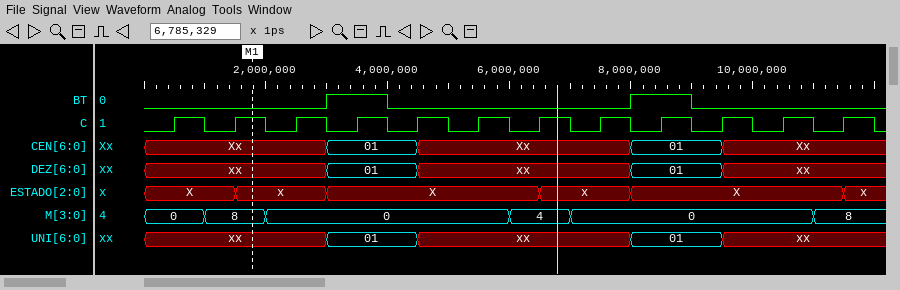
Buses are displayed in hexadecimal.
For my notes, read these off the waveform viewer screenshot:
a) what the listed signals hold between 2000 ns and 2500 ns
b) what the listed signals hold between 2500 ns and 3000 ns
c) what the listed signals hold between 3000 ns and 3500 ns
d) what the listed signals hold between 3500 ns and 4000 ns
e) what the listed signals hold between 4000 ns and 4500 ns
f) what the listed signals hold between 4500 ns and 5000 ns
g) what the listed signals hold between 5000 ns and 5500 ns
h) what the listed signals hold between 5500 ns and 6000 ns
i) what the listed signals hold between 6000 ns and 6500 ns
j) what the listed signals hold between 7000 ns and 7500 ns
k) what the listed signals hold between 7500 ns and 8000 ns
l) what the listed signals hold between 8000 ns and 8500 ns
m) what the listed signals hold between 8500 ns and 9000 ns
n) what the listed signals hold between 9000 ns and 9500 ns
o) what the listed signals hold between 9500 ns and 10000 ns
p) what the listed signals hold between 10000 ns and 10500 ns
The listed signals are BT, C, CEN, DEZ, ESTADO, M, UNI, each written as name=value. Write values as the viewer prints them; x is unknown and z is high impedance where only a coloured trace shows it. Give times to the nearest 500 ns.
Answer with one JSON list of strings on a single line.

["BT=0, C=0, CEN=Xx, DEZ=xx, ESTADO=x, M=0, UNI=xx", "BT=0, C=1, CEN=Xx, DEZ=xx, ESTADO=x, M=0, UNI=xx", "BT=1, C=0, CEN=01, DEZ=01, ESTADO=X, M=0, UNI=01", "BT=1, C=1, CEN=01, DEZ=01, ESTADO=X, M=0, UNI=01", "BT=0, C=0, CEN=01, DEZ=01, ESTADO=X, M=0, UNI=01", "BT=0, C=1, CEN=Xx, DEZ=xx, ESTADO=X, M=0, UNI=xx", "BT=0, C=0, CEN=Xx, DEZ=xx, ESTADO=X, M=0, UNI=xx", "BT=0, C=1, CEN=Xx, DEZ=xx, ESTADO=X, M=0, UNI=xx", "BT=0, C=0, CEN=Xx, DEZ=xx, ESTADO=X, M=4, UNI=xx", "BT=0, C=0, CEN=Xx, DEZ=xx, ESTADO=x, M=0, UNI=xx", "BT=0, C=1, CEN=Xx, DEZ=xx, ESTADO=x, M=0, UNI=xx", "BT=1, C=0, CEN=01, DEZ=01, ESTADO=X, M=0, UNI=01", "BT=1, C=1, CEN=01, DEZ=01, ESTADO=X, M=0, UNI=01", "BT=0, C=0, CEN=01, DEZ=01, ESTADO=X, M=0, UNI=01", "BT=0, C=1, CEN=Xx, DEZ=xx, ESTADO=X, M=0, UNI=xx", "BT=0, C=0, CEN=Xx, DEZ=xx, ESTADO=X, M=0, UNI=xx"]
